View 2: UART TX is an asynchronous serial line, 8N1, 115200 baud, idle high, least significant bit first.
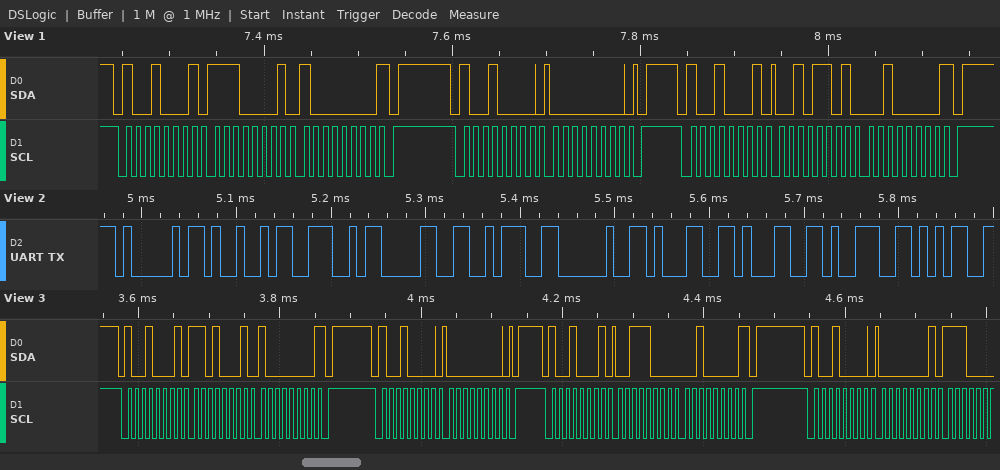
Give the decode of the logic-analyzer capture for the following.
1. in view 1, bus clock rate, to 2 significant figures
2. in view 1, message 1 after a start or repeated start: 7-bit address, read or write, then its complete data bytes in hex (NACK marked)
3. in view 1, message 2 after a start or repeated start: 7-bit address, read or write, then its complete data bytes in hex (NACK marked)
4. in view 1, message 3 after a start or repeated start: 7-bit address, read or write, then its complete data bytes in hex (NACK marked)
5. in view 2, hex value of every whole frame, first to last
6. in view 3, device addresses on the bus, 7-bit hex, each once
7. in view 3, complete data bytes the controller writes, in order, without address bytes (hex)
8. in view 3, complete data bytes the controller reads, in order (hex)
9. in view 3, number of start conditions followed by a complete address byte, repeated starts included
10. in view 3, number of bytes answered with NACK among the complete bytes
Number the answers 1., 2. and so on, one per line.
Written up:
1. 100 kHz
2. 0x48 read: E1 80 NACK
3. 0x48 write: 00
4. 0x48 read: 2D 20 NACK
5. 0x41 0x49 0x4E 0x30 0x3A 0x20 0x31 0x31 0x39 0x35
6. 0x48
7. 00 01
8. D1 80 38 20
9. 4
10. 2
